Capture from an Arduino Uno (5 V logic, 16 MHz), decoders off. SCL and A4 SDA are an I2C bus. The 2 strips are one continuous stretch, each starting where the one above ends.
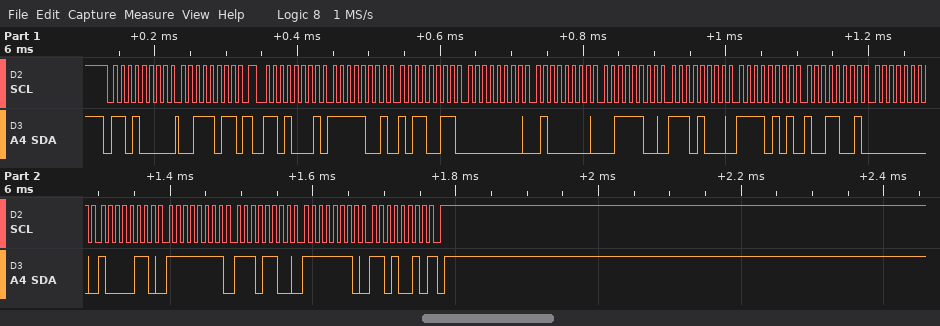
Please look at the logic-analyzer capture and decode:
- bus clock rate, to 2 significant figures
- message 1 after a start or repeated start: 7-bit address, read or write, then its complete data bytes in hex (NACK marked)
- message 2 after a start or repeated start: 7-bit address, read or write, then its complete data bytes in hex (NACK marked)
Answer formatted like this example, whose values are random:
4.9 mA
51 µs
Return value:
100 kHz
0x68 write: 3B
0x68 read: F9 B3 00 40 3C E8 F5 99 00 86 FF EC FE D2 NACK
